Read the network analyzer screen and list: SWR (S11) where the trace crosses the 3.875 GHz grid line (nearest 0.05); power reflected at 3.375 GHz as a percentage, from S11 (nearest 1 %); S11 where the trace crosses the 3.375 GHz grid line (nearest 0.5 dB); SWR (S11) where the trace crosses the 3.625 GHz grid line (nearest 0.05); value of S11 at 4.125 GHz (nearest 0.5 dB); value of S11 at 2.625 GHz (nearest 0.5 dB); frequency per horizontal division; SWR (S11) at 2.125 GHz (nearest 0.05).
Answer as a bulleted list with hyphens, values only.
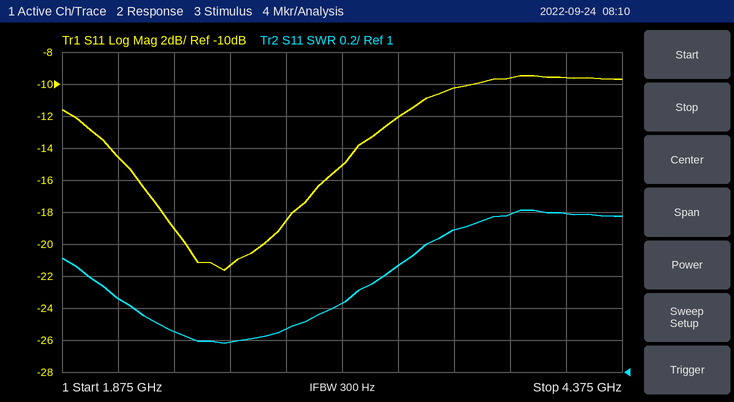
- 2.00
- 6 %
- -12.0 dB
- 1.90
- -9.5 dB
- -21.5 dB
- 250 MHz
- 1.45
